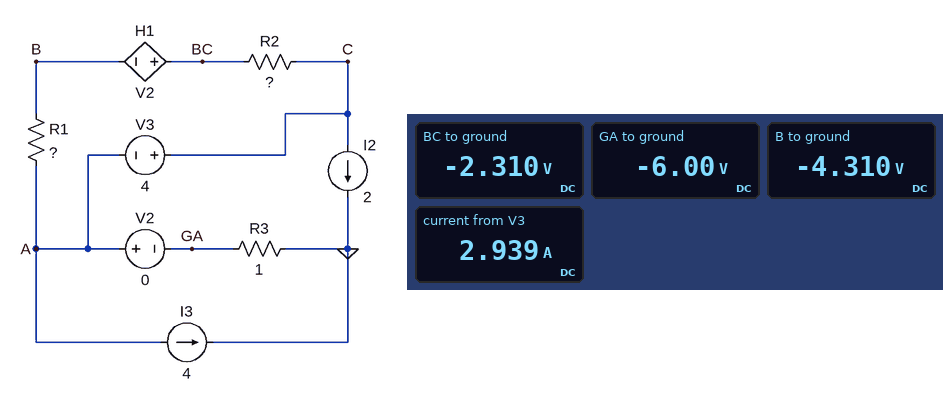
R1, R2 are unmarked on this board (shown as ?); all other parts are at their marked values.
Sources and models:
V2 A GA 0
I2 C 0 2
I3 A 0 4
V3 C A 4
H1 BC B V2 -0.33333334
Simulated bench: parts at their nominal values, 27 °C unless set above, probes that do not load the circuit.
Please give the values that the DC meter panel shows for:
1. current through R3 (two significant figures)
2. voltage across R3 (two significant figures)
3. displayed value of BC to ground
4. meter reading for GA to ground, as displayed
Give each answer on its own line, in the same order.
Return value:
6.0 A
6.0 V
-2.310 V
-6.00 V
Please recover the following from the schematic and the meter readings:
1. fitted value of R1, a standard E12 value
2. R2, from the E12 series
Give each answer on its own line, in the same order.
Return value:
1.8 Ω
0.33 Ω
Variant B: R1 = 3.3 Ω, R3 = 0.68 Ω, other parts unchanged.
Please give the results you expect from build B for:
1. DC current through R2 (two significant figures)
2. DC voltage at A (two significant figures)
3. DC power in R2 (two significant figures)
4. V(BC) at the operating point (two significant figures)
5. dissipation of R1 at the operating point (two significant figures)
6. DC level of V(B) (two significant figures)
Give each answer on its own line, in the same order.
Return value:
550 mA
-4.1 V
100 mW
-260 mV
1.0 W
-2.3 V
